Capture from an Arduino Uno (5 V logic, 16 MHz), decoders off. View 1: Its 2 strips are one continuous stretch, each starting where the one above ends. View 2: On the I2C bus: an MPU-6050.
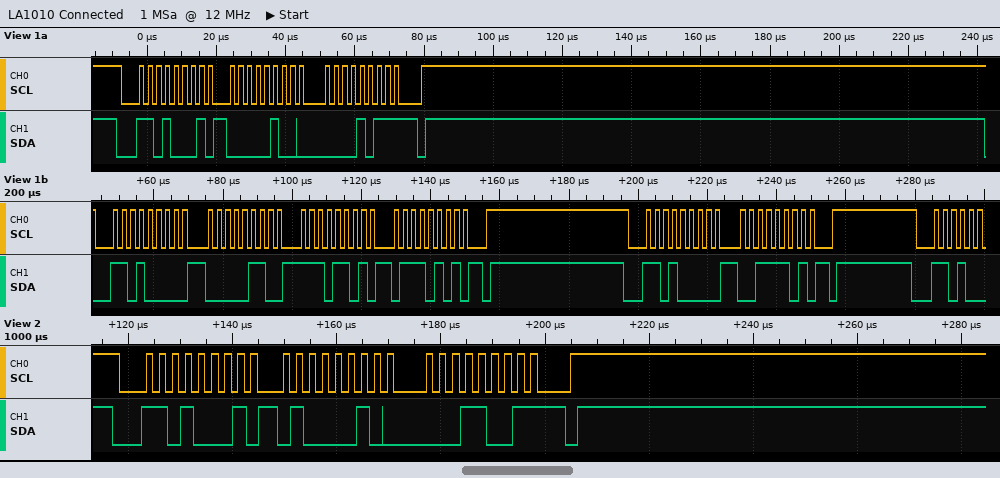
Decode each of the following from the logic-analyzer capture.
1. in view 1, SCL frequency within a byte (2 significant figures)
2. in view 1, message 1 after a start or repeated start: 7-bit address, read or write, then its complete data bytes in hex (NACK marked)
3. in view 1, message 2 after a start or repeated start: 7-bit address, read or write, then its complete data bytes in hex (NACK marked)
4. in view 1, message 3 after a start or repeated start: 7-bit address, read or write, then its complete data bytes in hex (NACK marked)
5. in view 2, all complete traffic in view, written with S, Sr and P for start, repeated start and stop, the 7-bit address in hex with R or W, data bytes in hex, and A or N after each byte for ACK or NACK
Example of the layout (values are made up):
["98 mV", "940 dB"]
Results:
["400 kHz", "0x68 read: 04 0B NACK", "0x68 write: 06 ED 75", "0x68 write: 3D", "S 68R A 42 A 19 N P"]
